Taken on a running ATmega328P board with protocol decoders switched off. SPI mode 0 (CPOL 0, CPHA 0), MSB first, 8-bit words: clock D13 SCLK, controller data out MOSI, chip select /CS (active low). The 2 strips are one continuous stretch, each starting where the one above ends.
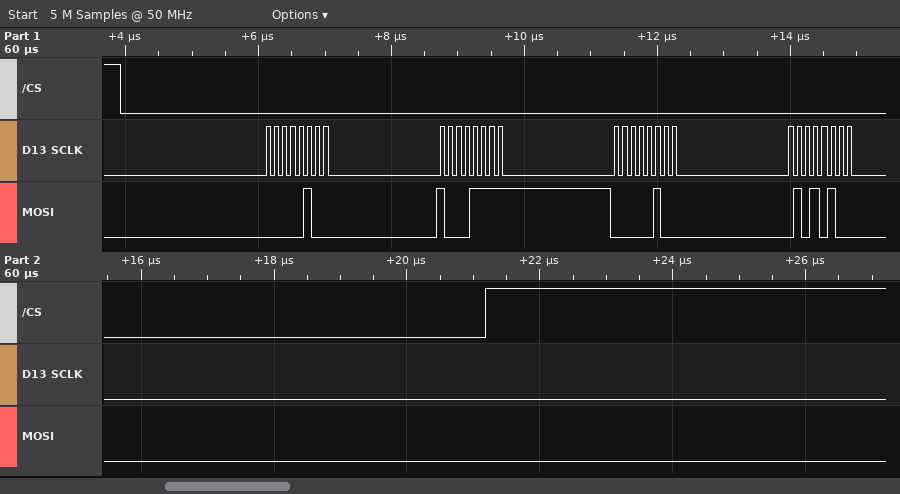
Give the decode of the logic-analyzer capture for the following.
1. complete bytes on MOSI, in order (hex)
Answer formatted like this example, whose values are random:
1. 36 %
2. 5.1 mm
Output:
1. 04 8F 04 54
